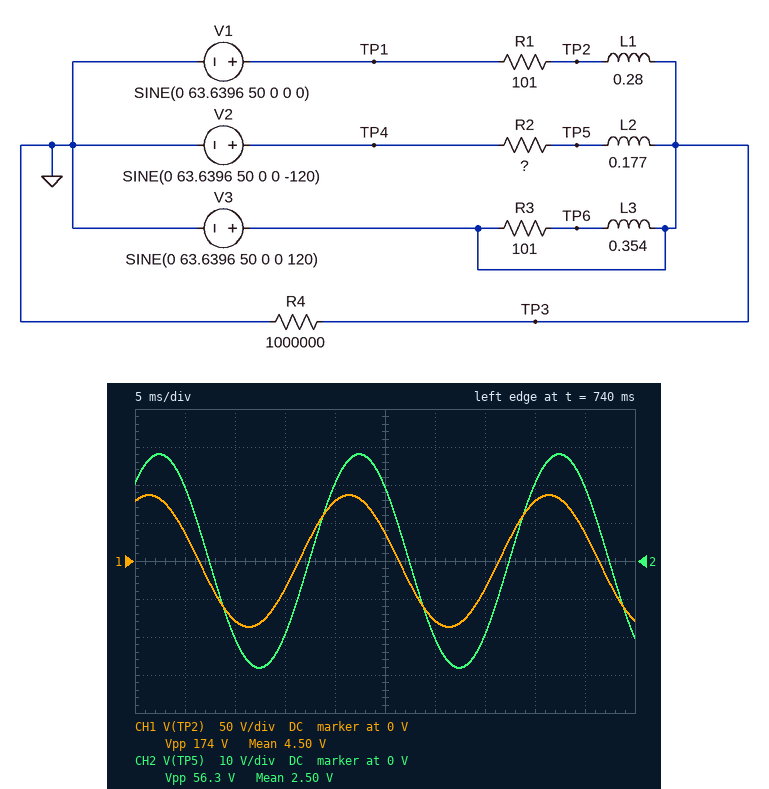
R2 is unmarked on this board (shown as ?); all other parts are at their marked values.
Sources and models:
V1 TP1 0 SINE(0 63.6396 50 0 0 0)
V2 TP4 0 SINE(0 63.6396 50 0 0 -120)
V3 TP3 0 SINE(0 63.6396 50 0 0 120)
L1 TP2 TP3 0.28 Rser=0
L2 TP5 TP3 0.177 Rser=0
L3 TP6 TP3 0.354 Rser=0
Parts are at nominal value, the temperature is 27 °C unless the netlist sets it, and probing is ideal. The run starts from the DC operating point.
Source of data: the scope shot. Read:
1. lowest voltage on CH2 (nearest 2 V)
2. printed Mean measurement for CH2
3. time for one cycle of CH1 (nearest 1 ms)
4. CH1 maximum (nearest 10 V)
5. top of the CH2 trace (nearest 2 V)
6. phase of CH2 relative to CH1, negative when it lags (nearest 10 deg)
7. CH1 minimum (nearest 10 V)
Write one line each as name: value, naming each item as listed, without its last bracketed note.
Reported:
lowest voltage on CH2: -28 V
printed Mean measurement for CH2: 2.50 V
time for one cycle of CH1: 20 ms
CH1 maximum: 90 V
top of the CH2 trace: 28 V
phase of CH2 relative to CH1, negative when it lags: -20 deg
CH1 minimum: -90 V
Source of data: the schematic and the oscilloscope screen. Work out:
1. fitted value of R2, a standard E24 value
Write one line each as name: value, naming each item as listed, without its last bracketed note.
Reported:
fitted value of R2, a standard E24 value: 82 Ω
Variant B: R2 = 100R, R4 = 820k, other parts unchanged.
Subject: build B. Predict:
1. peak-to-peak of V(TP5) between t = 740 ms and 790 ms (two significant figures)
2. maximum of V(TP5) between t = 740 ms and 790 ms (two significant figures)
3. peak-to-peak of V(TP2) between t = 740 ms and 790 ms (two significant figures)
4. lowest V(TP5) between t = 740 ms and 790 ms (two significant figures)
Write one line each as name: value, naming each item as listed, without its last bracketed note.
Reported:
peak-to-peak of V(TP5) between t = 740 ms and 790 ms: 65 V
maximum of V(TP5) between t = 740 ms and 790 ms: 33 V
peak-to-peak of V(TP2) between t = 740 ms and 790 ms: 170 V
lowest V(TP5) between t = 740 ms and 790 ms: -33 V
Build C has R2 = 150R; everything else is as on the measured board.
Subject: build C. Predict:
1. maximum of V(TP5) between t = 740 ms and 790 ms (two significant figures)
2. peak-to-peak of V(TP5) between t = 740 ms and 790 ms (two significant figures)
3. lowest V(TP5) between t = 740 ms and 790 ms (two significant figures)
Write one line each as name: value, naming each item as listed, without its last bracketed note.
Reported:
maximum of V(TP5) between t = 740 ms and 790 ms: 42 V
peak-to-peak of V(TP5) between t = 740 ms and 790 ms: 84 V
lowest V(TP5) between t = 740 ms and 790 ms: -42 V
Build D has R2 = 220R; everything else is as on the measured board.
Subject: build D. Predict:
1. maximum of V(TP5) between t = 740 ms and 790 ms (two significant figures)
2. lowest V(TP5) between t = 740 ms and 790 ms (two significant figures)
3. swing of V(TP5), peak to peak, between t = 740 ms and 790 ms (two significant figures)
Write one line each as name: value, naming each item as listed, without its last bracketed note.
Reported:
maximum of V(TP5) between t = 740 ms and 790 ms: 49 V
lowest V(TP5) between t = 740 ms and 790 ms: -49 V
swing of V(TP5), peak to peak, between t = 740 ms and 790 ms: 98 V
